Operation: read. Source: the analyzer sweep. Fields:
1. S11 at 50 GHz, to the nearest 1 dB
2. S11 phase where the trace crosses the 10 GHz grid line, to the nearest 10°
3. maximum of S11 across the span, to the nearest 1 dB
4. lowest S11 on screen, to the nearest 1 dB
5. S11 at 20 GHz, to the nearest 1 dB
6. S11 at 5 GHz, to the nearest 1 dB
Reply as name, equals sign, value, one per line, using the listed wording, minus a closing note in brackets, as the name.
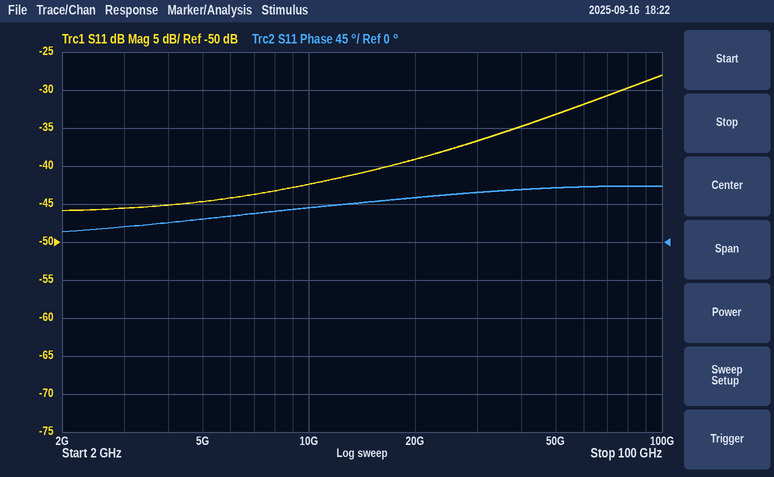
S11 at 50 GHz, to the nearest 1 dB = -33 dB
S11 phase where the trace crosses the 10 GHz grid line, to the nearest 10° = 40°
maximum of S11 across the span, to the nearest 1 dB = -28 dB
lowest S11 on screen, to the nearest 1 dB = -46 dB
S11 at 20 GHz, to the nearest 1 dB = -39 dB
S11 at 5 GHz, to the nearest 1 dB = -45 dB
